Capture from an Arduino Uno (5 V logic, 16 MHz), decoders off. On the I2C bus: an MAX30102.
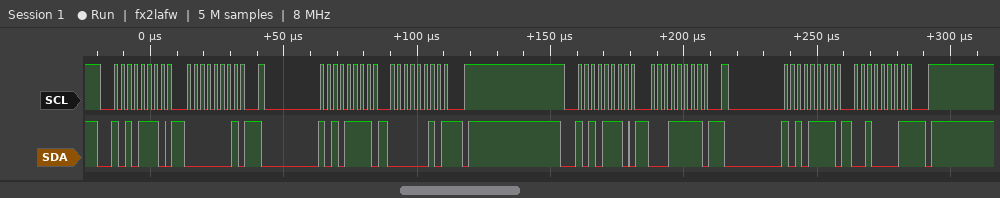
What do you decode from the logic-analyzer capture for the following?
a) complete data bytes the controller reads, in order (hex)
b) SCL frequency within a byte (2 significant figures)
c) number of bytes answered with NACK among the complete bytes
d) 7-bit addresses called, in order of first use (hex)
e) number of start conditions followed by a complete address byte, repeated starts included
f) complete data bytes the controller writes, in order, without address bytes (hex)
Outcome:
02 21
400 kHz
2
0x57
4
01 1F
